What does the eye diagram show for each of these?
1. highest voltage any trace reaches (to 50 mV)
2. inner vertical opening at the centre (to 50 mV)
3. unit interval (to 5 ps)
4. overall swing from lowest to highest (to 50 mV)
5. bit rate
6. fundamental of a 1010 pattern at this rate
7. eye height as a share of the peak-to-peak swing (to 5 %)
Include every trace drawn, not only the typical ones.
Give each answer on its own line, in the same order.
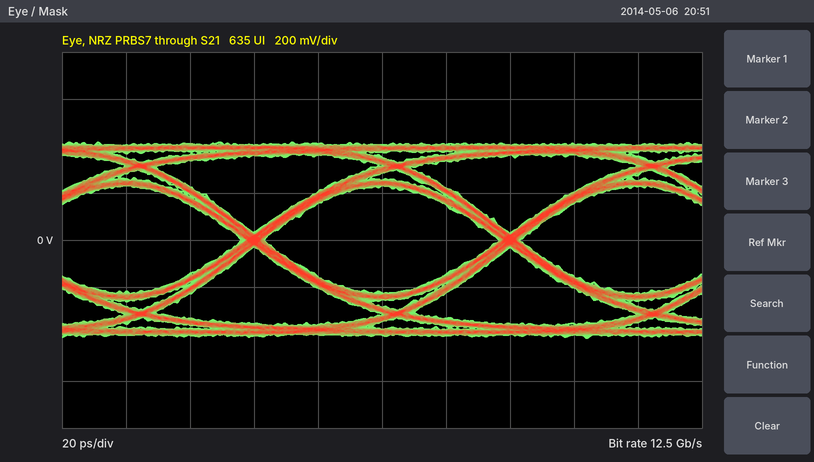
400 mV
450 mV
80 ps
850 mV
12.5 Gb/s
6.25 GHz
55 %
